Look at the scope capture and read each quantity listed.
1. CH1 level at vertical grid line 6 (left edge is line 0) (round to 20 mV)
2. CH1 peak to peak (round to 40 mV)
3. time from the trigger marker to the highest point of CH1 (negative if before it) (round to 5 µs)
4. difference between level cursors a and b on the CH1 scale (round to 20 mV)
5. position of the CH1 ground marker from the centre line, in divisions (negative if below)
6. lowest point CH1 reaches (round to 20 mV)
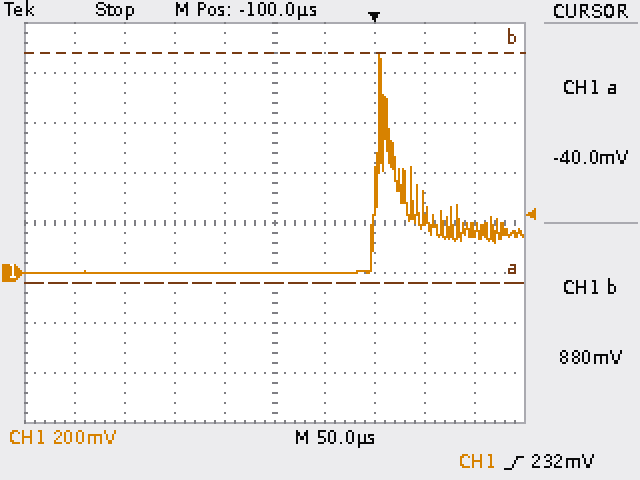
0 mV
880 mV
+5 µs
920 mV
-1.0 div
0 mV
